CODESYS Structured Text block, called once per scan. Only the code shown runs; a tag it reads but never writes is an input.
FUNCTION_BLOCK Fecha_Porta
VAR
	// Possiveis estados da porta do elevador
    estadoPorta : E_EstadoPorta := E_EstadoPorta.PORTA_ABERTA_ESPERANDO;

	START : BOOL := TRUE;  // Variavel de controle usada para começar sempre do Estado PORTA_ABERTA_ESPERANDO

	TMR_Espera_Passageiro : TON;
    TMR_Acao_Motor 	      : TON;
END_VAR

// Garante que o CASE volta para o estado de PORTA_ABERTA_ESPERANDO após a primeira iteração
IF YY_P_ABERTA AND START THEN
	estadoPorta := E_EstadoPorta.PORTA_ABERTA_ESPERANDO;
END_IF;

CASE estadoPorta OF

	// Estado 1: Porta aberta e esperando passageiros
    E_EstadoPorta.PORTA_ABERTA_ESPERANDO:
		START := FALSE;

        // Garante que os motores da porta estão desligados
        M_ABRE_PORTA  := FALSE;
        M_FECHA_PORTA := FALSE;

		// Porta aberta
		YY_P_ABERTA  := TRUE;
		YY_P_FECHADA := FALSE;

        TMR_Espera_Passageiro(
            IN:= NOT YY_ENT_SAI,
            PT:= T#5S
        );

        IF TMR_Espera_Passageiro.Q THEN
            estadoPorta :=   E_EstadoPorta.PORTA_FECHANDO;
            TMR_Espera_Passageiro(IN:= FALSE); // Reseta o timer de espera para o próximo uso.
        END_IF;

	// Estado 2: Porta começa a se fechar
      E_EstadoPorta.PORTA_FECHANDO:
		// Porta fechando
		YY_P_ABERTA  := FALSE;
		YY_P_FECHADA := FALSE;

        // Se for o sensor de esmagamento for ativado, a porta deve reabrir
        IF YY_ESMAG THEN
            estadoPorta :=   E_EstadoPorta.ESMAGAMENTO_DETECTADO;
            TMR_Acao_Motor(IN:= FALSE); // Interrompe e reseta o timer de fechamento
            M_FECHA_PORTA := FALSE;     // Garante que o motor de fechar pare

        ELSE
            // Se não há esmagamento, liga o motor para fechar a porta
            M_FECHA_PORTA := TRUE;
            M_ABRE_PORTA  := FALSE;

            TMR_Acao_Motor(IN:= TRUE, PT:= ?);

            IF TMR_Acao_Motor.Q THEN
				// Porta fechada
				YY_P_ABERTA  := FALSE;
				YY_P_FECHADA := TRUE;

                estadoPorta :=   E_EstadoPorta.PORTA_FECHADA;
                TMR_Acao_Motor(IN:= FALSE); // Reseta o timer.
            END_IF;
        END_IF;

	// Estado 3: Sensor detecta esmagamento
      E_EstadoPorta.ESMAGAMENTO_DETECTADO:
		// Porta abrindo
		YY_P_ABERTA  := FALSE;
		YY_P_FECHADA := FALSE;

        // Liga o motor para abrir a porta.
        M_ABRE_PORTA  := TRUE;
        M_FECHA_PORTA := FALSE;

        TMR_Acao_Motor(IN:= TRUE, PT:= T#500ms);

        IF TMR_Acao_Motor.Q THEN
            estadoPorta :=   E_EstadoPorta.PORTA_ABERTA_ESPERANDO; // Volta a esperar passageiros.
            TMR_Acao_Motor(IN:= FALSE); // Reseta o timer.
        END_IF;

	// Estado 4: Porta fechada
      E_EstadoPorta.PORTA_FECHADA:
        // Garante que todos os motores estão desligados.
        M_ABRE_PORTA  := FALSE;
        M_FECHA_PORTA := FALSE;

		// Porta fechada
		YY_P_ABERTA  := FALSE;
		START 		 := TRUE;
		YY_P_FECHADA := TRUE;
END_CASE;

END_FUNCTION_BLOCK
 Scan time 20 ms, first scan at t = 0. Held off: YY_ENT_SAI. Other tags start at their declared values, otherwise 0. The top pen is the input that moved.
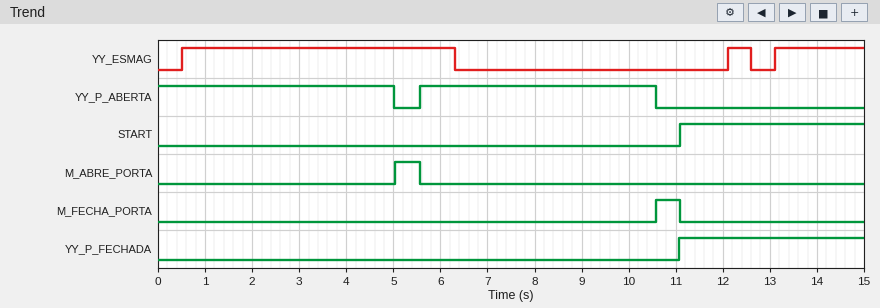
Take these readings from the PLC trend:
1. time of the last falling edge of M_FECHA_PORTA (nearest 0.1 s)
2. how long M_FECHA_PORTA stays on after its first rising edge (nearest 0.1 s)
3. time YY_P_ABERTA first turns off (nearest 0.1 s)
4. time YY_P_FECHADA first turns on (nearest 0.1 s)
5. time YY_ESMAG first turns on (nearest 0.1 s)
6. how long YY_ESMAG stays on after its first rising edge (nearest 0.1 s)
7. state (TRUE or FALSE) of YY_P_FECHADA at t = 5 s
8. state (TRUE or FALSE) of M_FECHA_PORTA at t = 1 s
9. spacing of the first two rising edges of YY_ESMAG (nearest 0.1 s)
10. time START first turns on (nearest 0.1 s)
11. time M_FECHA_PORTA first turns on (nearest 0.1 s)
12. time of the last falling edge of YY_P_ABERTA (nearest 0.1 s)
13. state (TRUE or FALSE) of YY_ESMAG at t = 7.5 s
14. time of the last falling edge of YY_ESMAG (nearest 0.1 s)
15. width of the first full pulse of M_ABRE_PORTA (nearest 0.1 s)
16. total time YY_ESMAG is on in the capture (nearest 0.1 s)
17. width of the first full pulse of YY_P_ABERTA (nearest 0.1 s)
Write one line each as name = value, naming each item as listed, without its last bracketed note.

time of the last falling edge of M_FECHA_PORTA = 11.1 s
how long M_FECHA_PORTA stays on after its first rising edge = 0.5 s
time YY_P_ABERTA first turns off = 5.0 s
time YY_P_FECHADA first turns on = 11.1 s
time YY_ESMAG first turns on = 0.5 s
how long YY_ESMAG stays on after its first rising edge = 5.8 s
state (TRUE or FALSE) of YY_P_FECHADA at t = 5 s = FALSE
state (TRUE or FALSE) of M_FECHA_PORTA at t = 1 s = FALSE
spacing of the first two rising edges of YY_ESMAG = 11.6 s
time START first turns on = 11.1 s
time M_FECHA_PORTA first turns on = 10.6 s
time of the last falling edge of YY_P_ABERTA = 10.6 s
state (TRUE or FALSE) of YY_ESMAG at t = 7.5 s = FALSE
time of the last falling edge of YY_ESMAG = 12.6 s
width of the first full pulse of M_ABRE_PORTA = 0.5 s
total time YY_ESMAG is on in the capture = 8.2 s
width of the first full pulse of YY_P_ABERTA = 5.0 s
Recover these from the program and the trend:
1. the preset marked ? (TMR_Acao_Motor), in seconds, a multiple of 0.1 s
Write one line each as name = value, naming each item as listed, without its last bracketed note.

the preset marked ? (TMR_Acao_Motor), in seconds, a multiple of 0.1 s = 0.5 s
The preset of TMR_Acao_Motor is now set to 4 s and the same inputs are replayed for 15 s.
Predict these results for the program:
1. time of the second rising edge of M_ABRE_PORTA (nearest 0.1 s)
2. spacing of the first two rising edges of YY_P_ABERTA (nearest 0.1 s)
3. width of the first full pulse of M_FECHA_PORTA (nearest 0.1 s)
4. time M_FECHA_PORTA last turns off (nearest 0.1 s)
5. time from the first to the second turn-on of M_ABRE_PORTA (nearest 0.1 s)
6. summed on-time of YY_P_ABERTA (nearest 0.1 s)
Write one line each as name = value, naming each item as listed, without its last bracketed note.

time of the second rising edge of M_ABRE_PORTA = 12.1 s
spacing of the first two rising edges of YY_P_ABERTA = 7.1 s
width of the first full pulse of M_FECHA_PORTA = 1.5 s
time M_FECHA_PORTA last turns off = 12.1 s
time from the first to the second turn-on of M_ABRE_PORTA = 7.1 s
summed on-time of YY_P_ABERTA = 12.4 s
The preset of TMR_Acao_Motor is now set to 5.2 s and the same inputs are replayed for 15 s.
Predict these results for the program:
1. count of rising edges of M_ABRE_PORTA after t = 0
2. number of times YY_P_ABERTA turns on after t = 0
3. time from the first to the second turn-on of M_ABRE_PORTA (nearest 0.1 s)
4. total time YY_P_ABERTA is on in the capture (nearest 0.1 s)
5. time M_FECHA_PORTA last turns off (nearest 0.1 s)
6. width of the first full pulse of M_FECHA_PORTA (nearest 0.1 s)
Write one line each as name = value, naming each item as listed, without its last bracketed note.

count of rising edges of M_ABRE_PORTA after t = 0 = 2
number of times YY_P_ABERTA turns on after t = 0 = 2
time from the first to the second turn-on of M_ABRE_PORTA = 7.1 s
total time YY_P_ABERTA is on in the capture = 12.4 s
time M_FECHA_PORTA last turns off = 12.1 s
width of the first full pulse of M_FECHA_PORTA = 1.5 s
